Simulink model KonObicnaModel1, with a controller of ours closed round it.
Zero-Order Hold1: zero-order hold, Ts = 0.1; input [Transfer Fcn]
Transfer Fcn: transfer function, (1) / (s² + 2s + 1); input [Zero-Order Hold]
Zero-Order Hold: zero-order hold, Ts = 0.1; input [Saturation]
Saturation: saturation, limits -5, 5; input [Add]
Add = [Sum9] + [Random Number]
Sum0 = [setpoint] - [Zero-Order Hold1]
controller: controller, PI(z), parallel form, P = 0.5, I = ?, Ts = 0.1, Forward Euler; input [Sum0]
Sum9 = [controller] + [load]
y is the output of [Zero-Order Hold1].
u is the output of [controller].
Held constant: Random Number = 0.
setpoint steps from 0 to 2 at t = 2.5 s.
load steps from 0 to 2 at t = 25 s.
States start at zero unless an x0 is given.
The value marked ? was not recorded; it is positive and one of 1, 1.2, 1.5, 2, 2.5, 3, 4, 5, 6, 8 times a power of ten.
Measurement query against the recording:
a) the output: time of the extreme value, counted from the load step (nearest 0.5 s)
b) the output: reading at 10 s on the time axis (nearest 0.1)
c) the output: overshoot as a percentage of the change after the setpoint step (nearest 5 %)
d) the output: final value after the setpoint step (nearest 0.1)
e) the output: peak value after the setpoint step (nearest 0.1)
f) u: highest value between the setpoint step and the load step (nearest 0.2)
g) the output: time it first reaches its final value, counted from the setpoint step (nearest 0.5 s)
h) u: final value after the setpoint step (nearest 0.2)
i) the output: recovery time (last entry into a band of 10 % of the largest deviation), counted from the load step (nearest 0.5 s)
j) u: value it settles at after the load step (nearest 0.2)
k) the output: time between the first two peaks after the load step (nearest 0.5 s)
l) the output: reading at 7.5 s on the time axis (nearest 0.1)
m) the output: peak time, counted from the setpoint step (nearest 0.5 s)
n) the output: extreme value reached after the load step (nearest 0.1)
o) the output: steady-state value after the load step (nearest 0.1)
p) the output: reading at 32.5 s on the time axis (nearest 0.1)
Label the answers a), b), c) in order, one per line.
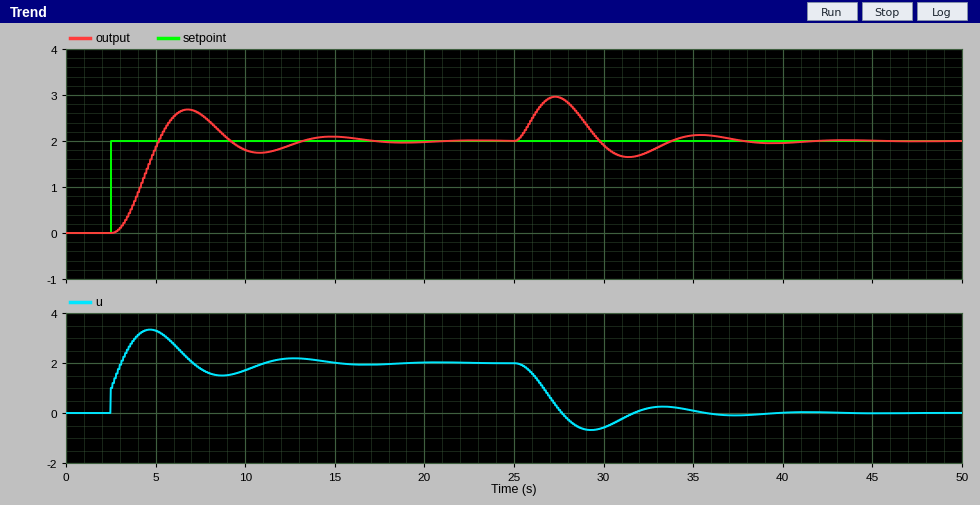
a) 2.5 s
b) 1.8
c) 35 %
d) 2.0
e) 2.7
f) 3.4
g) 2.5 s
h) 2.0
i) 11.5 s
j) 0.0
k) 8.0 s
l) 2.6
m) 4.5 s
n) 3.0
o) 2.0
p) 1.8
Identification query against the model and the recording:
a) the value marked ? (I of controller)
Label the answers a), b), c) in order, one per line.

a) 1
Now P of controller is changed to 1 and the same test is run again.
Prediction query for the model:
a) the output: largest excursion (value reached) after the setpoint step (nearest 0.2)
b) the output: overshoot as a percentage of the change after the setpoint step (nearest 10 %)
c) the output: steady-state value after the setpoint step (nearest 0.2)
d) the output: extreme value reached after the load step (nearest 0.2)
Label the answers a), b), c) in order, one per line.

a) 2.4
b) 20 %
c) 2.0
d) 2.8
